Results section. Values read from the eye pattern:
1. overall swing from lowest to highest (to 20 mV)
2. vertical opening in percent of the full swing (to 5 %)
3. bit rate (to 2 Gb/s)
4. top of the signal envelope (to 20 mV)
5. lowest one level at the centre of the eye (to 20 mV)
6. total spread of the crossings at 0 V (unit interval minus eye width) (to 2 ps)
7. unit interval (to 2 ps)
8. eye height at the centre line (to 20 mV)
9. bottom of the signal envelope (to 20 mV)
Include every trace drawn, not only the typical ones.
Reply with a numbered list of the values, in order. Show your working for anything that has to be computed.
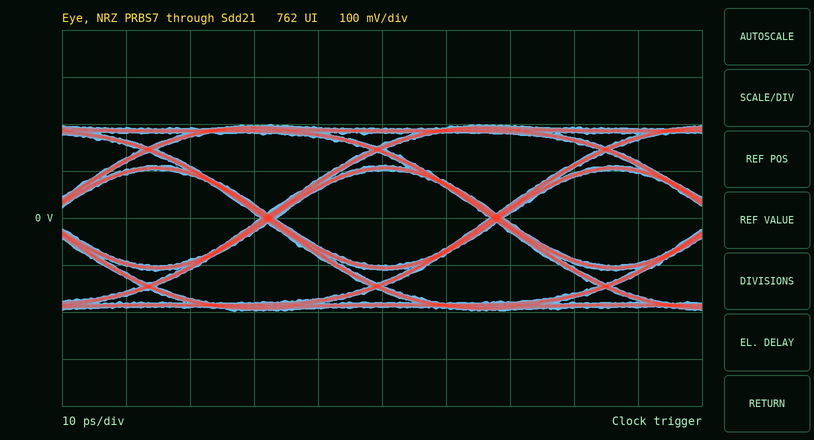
1. 400 mV
2. 200 mV / 400 mV ≈ 50 %
3. 28 Gb/s
4. 200 mV
5. 100 mV
6. 2 ps
7. 36 ps
8. 200 mV
9. -200 mV
